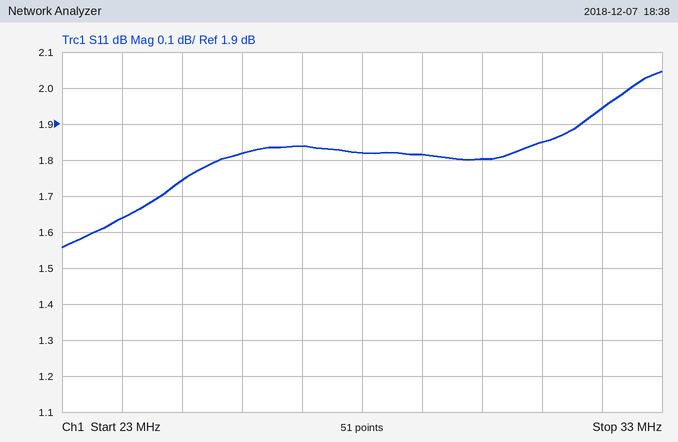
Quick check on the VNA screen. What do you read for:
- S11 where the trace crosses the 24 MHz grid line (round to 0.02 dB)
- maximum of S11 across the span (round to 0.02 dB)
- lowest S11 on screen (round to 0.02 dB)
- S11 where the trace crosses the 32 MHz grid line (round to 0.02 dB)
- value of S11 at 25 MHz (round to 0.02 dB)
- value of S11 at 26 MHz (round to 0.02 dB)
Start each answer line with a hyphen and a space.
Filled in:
- 1.64 dB
- 2.04 dB
- 1.56 dB
- 1.94 dB
- 1.74 dB
- 1.82 dB
